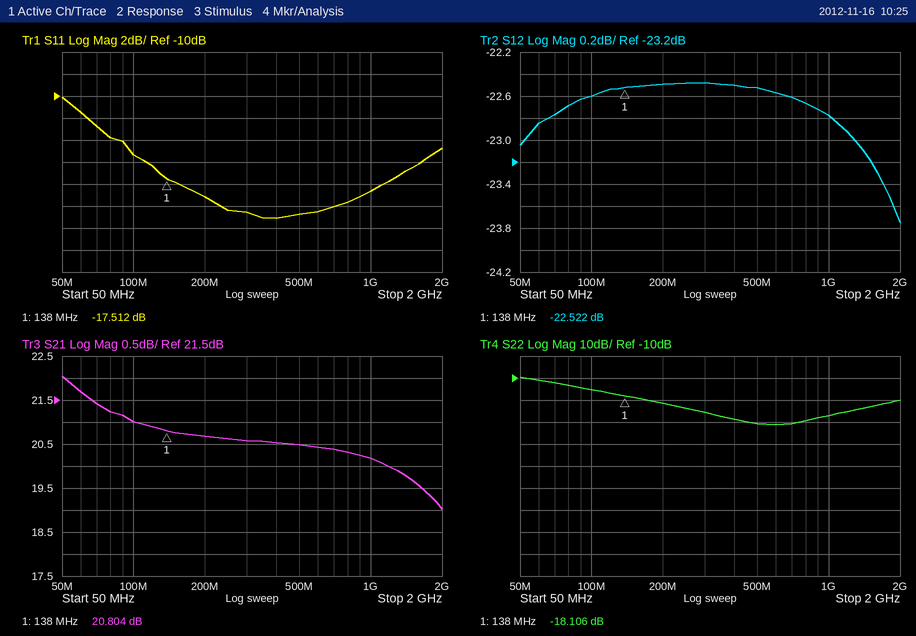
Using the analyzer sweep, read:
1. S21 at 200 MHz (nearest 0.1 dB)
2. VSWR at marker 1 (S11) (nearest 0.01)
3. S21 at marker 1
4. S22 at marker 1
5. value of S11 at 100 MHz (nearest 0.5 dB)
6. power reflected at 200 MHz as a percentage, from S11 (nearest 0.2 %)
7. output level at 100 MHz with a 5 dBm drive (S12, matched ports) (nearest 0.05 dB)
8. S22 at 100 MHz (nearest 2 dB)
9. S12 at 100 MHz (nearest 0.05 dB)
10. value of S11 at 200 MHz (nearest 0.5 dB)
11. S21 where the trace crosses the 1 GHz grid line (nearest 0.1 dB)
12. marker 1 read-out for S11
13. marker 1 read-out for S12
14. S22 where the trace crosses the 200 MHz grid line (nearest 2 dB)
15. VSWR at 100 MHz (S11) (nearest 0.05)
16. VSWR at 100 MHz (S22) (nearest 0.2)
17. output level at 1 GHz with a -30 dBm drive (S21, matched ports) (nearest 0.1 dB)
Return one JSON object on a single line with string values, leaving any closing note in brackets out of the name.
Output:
{"S21 at 200 MHz": "20.7 dB", "VSWR at marker 1 (S11)": "1.31", "S21 at marker 1": "20.804 dB", "S22 at marker 1": "-18.106 dB", "value of S11 at 100 MHz": "-15.5 dB", "power reflected at 200 MHz as a percentage, from S11": "1.2 %", "output level at 100 MHz with a 5 dBm drive (S12, matched ports)": "-17.60 dBm", "S22 at 100 MHz": "-16 dB", "S12 at 100 MHz": "-22.60 dB", "value of S11 at 200 MHz": "-19.0 dB", "S21 where the trace crosses the 1 GHz grid line": "20.2 dB", "marker 1 read-out for S11": "-17.512 dB", "marker 1 read-out for S12": "-22.522 dB", "S22 where the trace crosses the 200 MHz grid line": "-22 dB", "VSWR at 100 MHz (S11)": "1.40", "VSWR at 100 MHz (S22)": "1.4", "output level at 1 GHz with a -30 dBm drive (S21, matched ports)": "-9.8 dBm"}
